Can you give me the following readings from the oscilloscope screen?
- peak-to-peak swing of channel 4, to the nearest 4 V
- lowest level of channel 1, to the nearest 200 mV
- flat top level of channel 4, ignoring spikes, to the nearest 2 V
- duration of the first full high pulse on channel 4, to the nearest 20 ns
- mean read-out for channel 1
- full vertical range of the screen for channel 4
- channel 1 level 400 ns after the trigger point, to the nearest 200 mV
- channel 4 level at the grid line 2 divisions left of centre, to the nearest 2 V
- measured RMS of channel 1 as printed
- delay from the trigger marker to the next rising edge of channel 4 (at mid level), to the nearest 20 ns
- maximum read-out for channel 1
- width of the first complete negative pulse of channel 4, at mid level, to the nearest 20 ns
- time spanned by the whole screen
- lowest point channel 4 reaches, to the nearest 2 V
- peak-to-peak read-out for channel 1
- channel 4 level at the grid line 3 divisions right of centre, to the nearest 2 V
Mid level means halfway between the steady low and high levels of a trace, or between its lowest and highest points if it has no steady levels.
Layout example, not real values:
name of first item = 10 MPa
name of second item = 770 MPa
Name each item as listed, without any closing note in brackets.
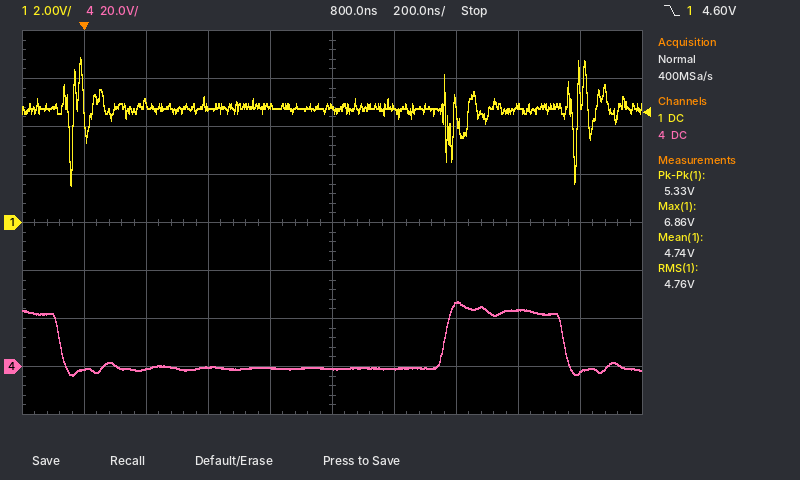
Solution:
peak-to-peak swing of channel 4, to the nearest 4 V = 32 V
lowest level of channel 1, to the nearest 200 mV = 1.6 V
flat top level of channel 4, ignoring spikes, to the nearest 2 V = 22 V
duration of the first full high pulse on channel 4, to the nearest 20 ns = 380 ns
mean read-out for channel 1 = 4.74 V
full vertical range of the screen for channel 4 = 160 V
channel 1 level 400 ns after the trigger point, to the nearest 200 mV = 4.8 V
channel 4 level at the grid line 2 divisions left of centre, to the nearest 2 V = 0 V
measured RMS of channel 1 as printed = 4.76 V
delay from the trigger marker to the next rising edge of channel 4 (at mid level), to the nearest 20 ns = 1.16 µs
maximum read-out for channel 1 = 6.86 V
width of the first complete negative pulse of channel 4, at mid level, to the nearest 20 ns = 1.24 µs
time spanned by the whole screen = 2 µs
lowest point channel 4 reaches, to the nearest 2 V = -4 V
peak-to-peak read-out for channel 1 = 5.33 V
channel 4 level at the grid line 3 divisions right of centre, to the nearest 2 V = 24 V
